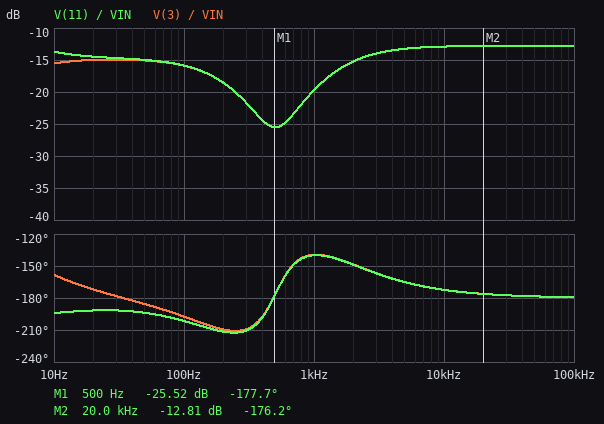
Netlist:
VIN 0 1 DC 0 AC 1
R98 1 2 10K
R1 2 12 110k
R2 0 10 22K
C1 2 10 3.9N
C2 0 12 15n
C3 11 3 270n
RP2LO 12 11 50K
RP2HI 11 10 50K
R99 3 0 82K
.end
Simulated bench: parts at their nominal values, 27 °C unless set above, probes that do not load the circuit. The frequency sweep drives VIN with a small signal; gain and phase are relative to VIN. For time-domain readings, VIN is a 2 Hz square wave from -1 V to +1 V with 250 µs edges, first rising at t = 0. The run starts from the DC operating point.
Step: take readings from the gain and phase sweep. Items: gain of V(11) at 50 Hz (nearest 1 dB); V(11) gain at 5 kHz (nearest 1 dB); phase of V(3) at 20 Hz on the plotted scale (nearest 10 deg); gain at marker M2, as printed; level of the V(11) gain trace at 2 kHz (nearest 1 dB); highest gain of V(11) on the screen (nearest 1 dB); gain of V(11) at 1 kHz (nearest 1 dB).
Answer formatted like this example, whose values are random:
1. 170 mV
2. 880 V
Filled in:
1. -15 dB
2. -13 dB
3. -170 deg
4. -12.81 dB
5. -15 dB
6. -13 dB
7. -20 dB
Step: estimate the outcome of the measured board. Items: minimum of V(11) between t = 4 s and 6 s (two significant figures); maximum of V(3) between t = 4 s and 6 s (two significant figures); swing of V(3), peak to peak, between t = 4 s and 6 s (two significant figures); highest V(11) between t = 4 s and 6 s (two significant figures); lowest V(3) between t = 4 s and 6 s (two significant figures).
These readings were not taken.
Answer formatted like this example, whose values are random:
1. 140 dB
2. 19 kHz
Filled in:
1. -300 mV
2. 340 mV
3. 670 mV
4. 300 mV
5. -340 mV
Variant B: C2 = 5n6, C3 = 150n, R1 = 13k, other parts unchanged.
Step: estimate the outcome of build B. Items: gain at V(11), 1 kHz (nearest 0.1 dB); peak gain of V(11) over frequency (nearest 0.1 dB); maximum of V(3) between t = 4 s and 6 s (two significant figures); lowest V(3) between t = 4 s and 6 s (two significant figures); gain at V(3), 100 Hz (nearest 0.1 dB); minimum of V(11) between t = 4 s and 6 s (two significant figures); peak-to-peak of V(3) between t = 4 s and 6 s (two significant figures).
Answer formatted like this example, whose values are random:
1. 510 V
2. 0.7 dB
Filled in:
1. -10.7 dB
2. -6.1 dB
3. 670 mV
4. -670 mV
5. -9.3 dB
6. -500 mV
7. 1.3 V
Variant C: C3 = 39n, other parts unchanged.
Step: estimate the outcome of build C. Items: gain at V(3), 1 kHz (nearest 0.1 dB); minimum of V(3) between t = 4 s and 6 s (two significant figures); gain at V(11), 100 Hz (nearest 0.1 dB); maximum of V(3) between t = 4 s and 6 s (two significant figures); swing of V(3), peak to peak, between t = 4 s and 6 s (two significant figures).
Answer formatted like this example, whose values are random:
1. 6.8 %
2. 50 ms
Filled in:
1. -19.7 dB
2. -250 mV
3. -15.5 dB
4. 250 mV
5. 510 mV
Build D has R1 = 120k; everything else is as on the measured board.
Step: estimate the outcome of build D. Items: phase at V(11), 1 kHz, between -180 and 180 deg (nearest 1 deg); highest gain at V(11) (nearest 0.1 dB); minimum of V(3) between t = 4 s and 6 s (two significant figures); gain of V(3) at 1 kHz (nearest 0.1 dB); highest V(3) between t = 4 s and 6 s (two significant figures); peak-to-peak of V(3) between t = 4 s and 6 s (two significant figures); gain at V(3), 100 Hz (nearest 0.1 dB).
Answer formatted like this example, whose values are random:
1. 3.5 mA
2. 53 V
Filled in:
1. -139 deg
2. -10.9 dB
3. -320 mV
4. -19.5 dB
5. 320 mV
6. 640 mV
7. -16.4 dB
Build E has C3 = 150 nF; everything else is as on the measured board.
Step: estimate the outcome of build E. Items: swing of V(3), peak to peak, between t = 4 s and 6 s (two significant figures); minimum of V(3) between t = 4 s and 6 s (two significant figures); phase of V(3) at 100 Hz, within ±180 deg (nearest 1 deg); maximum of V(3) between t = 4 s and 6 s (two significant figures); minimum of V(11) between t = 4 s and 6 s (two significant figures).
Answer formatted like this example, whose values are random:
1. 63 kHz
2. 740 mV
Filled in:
1. 640 mV
2. -320 mV
3. 165 deg
4. 320 mV
5. -300 mV
